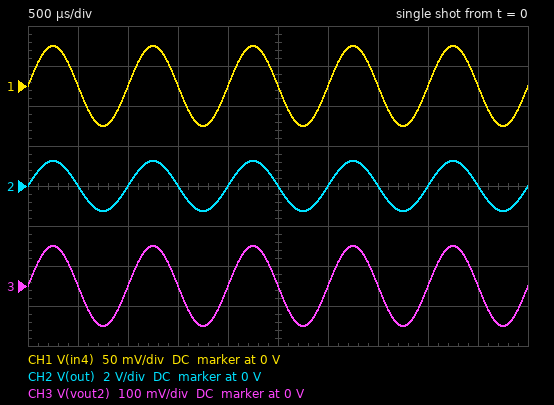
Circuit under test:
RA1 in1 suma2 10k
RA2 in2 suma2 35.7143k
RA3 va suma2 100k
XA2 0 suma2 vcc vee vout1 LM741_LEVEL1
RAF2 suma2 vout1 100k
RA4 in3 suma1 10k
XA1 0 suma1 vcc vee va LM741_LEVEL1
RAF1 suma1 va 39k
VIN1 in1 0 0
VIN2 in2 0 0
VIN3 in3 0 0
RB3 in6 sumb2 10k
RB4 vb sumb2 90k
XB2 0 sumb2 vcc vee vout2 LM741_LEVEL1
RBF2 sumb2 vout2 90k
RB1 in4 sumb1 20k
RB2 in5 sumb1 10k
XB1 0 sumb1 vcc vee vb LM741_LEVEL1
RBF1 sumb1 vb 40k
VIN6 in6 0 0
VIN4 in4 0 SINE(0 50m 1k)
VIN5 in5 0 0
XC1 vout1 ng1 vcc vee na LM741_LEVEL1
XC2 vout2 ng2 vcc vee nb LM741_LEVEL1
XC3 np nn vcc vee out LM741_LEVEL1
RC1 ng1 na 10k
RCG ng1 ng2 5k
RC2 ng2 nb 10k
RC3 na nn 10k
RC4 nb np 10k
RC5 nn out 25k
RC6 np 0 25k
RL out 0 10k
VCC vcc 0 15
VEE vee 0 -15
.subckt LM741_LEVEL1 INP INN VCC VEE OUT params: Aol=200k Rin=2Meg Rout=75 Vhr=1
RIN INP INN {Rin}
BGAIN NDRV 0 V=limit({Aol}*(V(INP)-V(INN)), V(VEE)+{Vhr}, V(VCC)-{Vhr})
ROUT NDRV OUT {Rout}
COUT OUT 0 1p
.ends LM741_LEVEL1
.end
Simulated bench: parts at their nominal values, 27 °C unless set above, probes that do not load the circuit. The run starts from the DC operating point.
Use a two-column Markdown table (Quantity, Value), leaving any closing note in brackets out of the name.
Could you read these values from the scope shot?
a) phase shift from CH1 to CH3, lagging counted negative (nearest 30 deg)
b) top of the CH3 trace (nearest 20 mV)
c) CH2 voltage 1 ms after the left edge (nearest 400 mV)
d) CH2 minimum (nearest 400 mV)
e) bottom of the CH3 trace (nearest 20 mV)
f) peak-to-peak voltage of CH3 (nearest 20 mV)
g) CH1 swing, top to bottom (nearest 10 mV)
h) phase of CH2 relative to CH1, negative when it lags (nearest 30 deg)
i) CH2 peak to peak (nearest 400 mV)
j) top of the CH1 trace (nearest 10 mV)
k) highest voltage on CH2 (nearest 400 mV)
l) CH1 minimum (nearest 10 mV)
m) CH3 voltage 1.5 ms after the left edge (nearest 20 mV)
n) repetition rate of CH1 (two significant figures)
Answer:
| Quantity | Value |
|---|---|
| phase shift from CH1 to CH3, lagging counted negative | 0 deg |
| top of the CH3 trace | 100 mV |
| CH2 voltage 1 ms after the left edge | 0 V |
| CH2 minimum | -1.2 V |
| bottom of the CH3 trace | -100 mV |
| peak-to-peak voltage of CH3 | 200 mV |
| CH1 swing, top to bottom | 100 mV |
| phase of CH2 relative to CH1, negative when it lags | 0 deg |
| CH2 peak to peak | 2.4 V |
| top of the CH1 trace | 50 mV |
| highest voltage on CH2 | 1.2 V |
| CH1 minimum | -50 mV |
| CH3 voltage 1.5 ms after the left edge | 0 V |
| repetition rate of CH1 | 1.0 kHz |
